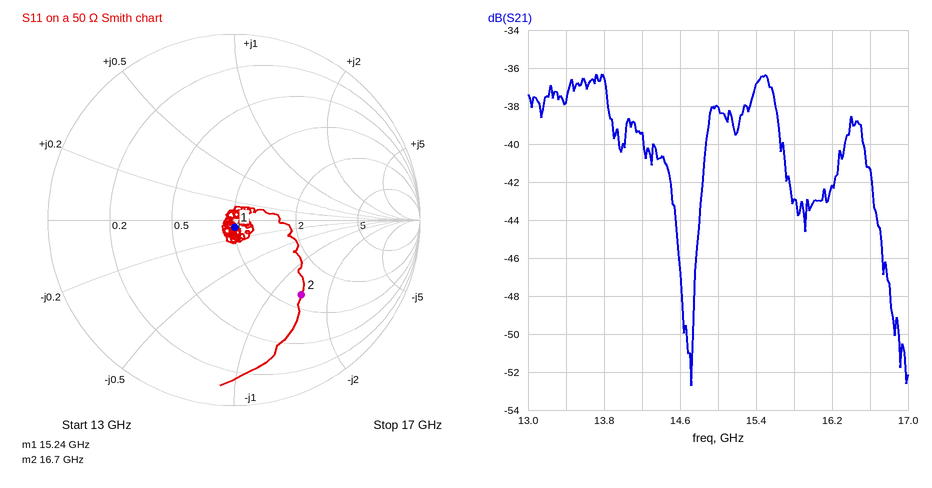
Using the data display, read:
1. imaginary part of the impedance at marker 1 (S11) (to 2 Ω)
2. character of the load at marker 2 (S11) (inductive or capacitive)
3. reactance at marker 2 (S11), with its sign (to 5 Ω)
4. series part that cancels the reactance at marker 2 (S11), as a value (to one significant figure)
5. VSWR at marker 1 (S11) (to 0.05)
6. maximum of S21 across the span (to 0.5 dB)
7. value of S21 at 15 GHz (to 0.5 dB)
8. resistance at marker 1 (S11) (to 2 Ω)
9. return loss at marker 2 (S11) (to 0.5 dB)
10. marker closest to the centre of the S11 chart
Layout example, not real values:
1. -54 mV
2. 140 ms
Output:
1. -4 Ω
2. capacitive
3. -70 Ω
4. 700 pH
5. 1.10
6. -36.5 dB
7. -38.0 dB
8. 50 Ω
9. 5.5 dB
10. marker 1
